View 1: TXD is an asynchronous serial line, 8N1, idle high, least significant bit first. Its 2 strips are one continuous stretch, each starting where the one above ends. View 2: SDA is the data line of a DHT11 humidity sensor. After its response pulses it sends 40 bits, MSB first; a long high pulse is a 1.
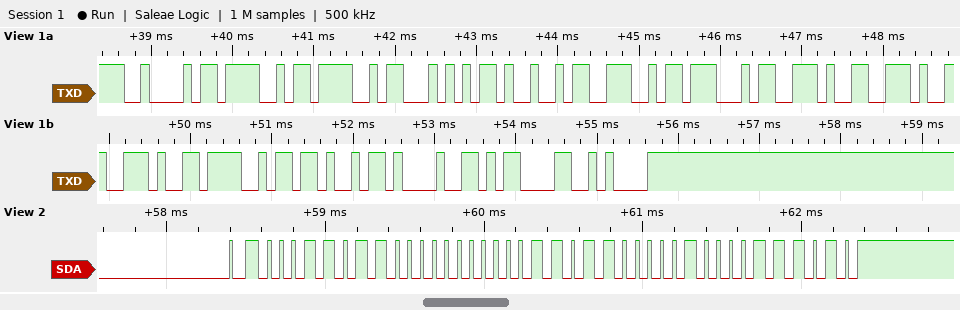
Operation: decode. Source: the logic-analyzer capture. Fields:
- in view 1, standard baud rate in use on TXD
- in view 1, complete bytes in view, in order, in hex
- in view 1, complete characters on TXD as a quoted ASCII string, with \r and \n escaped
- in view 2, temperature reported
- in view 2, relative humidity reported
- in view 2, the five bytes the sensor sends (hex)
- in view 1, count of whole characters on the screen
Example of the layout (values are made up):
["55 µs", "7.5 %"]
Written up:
["9600 baud", "42 4F 4F 54 49 4E 47 2E 2E 2E 4F 4B 21 0D 0A", "\"BOOTING...OK!\\r\\n\"", "27.4 °C", "27 %", "1B 00 1B 04 3A", "15"]
